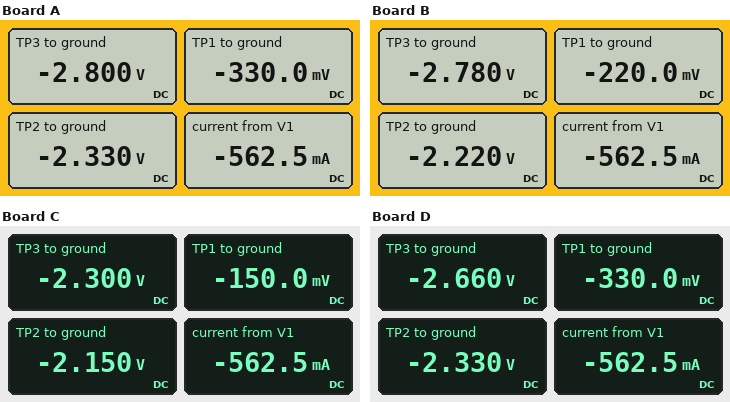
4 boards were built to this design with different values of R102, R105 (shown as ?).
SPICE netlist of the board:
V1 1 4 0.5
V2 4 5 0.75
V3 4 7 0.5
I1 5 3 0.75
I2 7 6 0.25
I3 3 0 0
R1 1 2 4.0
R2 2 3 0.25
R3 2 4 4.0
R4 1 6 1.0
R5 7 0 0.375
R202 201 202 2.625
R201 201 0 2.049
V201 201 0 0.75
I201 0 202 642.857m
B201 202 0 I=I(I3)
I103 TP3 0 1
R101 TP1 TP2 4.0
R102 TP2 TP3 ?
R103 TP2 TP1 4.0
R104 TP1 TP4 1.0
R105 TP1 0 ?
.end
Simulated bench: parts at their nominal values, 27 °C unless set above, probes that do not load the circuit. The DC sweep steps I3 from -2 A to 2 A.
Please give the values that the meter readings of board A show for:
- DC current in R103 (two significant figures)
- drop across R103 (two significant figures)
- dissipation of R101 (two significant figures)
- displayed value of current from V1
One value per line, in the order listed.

500 mA
2.0 V
1.0 W
-562.5 mA
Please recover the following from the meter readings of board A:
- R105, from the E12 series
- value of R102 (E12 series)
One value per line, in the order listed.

0.33 Ω
0.47 Ω
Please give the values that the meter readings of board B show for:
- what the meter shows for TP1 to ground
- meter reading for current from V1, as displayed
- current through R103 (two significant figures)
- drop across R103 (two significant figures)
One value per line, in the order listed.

-220.0 mV
-562.5 mA
500 mA
2.0 V
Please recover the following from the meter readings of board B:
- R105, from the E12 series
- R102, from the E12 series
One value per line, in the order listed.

0.22 Ω
0.56 Ω
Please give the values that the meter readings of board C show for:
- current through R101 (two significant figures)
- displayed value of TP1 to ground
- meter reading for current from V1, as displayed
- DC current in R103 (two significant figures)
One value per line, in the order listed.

500 mA
-150.0 mV
-562.5 mA
500 mA
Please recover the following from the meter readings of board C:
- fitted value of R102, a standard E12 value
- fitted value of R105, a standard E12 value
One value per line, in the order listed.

0.15 Ω
0.15 Ω
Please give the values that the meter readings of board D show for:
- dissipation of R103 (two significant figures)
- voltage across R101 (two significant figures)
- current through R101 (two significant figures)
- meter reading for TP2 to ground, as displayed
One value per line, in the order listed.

1.0 W
2.0 V
500 mA
-2.330 V
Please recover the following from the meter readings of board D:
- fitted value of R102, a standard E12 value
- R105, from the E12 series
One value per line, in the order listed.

0.33 Ω
0.33 Ω
